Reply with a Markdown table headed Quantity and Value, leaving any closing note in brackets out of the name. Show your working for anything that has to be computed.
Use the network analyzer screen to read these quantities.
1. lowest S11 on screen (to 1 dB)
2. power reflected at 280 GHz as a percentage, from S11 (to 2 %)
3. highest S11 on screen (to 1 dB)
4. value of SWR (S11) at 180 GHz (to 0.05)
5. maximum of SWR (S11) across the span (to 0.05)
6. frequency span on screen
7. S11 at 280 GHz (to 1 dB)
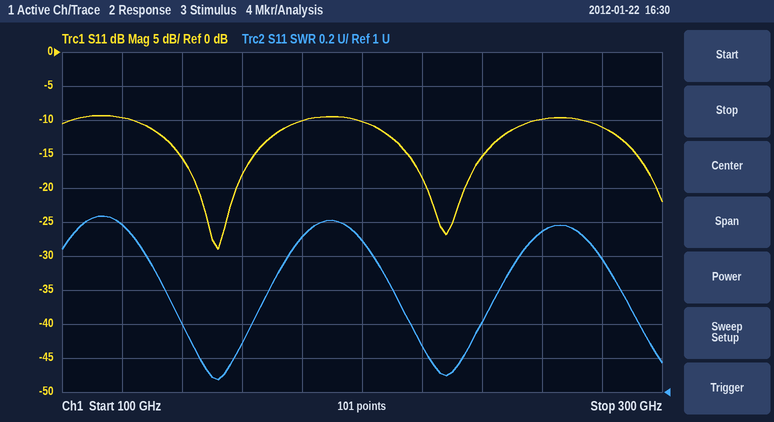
| Quantity | Value |
|---|---|
| lowest S11 on screen | -29 dB |
| power reflected at 280 GHz as a percentage, from S11 | 10^(-11/10) ≈ 8 % |
| highest S11 on screen | -9 dB |
| value of SWR (S11) at 180 GHz | 1.90 |
| maximum of SWR (S11) across the span | 2.05 |
| frequency span on screen | 200 GHz |
| S11 at 280 GHz | -11 dB |
